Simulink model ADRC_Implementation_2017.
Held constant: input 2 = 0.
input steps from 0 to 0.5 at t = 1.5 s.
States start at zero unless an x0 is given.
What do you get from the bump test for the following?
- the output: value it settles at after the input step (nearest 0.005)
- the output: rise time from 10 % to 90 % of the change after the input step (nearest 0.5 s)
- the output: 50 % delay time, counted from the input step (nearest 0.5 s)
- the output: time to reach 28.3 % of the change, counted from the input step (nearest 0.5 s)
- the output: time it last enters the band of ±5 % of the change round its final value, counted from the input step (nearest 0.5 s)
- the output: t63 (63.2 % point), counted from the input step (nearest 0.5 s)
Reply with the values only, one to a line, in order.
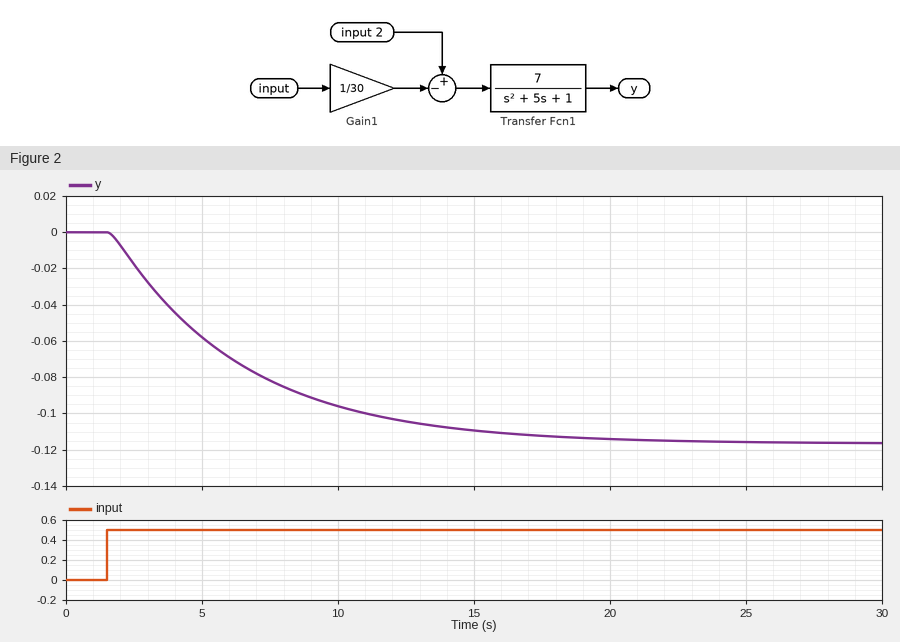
-0.115
10.5 s
3.5 s
2.0 s
14.5 s
5.0 s
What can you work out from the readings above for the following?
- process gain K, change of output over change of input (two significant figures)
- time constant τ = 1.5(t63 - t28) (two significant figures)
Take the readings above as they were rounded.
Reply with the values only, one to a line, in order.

-0.23
4.5 s
